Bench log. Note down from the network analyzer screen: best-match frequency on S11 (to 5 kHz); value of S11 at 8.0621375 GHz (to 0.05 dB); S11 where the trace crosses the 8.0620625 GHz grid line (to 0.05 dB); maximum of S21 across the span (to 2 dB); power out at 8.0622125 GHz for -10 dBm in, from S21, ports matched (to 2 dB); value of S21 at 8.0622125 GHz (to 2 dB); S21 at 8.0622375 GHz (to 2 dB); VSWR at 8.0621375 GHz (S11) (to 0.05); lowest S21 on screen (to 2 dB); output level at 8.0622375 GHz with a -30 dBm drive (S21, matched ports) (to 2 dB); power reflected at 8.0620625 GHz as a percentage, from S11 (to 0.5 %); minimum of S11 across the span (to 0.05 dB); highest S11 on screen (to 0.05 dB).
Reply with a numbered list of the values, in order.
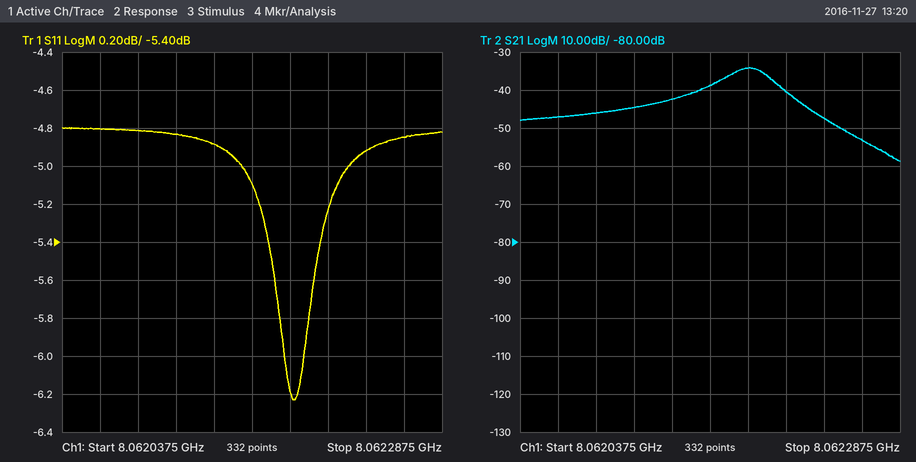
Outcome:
1. 8.062190 GHz
2. -4.90 dB
3. -4.80 dB
4. -34 dB
5. -50 dBm
6. -40 dB
7. -48 dB
8. 3.65
9. -58 dB
10. -78 dBm
11. 33.0 %
12. -6.25 dB
13. -4.80 dB
